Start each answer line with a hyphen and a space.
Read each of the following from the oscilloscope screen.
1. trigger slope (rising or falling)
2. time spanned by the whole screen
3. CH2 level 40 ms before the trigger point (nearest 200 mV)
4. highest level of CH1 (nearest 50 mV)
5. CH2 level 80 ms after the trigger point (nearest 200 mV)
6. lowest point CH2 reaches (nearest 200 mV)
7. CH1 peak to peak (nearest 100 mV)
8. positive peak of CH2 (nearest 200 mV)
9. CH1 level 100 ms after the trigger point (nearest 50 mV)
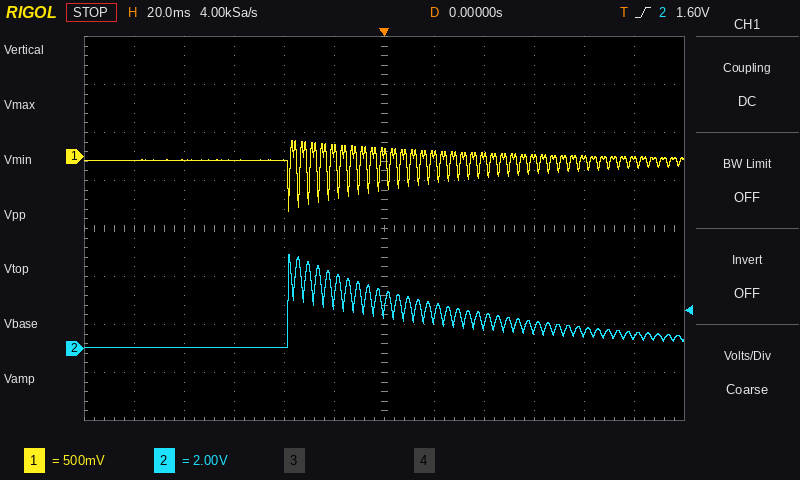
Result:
- rising
- 240 ms
- 0.0 V
- 150 mV
- 600 mV
- 0.0 V
- 700 mV
- 4.0 V
- -50 mV
